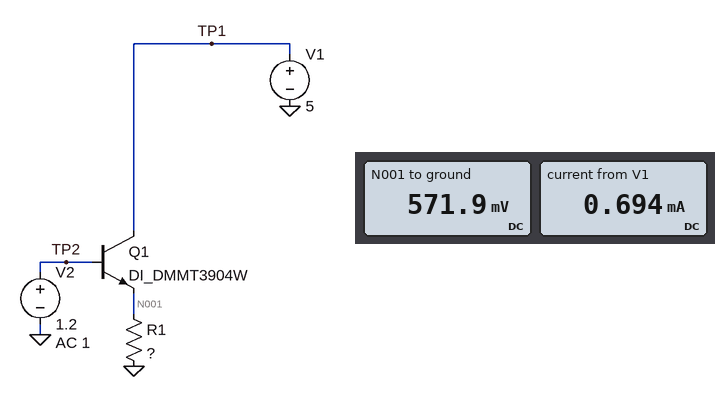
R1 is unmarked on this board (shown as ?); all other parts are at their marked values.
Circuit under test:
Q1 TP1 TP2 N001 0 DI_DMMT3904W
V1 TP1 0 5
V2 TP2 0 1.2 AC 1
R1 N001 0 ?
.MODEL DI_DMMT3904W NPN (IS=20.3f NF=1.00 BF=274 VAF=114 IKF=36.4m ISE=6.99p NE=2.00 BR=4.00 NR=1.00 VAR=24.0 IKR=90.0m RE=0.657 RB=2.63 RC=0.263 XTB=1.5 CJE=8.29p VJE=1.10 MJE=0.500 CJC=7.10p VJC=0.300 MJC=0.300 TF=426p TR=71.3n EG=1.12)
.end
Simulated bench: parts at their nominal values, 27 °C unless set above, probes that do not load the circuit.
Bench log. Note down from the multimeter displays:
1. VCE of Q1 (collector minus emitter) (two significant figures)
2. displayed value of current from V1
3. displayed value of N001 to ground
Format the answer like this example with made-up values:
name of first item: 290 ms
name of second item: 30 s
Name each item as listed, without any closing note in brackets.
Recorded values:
VCE of Q1 (collector minus emitter): 4.4 V
displayed value of current from V1: 0.694 mA
displayed value of N001 to ground: 571.9 mV
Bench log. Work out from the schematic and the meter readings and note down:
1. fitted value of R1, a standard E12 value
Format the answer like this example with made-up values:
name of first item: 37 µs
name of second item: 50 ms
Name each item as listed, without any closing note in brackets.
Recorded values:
fitted value of R1, a standard E12 value: 820 Ω
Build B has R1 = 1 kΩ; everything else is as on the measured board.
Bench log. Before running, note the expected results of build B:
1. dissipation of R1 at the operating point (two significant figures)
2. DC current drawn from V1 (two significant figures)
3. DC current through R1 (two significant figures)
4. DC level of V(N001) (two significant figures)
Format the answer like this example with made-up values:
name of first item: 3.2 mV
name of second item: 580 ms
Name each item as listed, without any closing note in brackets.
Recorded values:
dissipation of R1 at the operating point: 330 µW
DC current drawn from V1: 570 µA
DC current through R1: 580 µA
DC level of V(N001): 580 mV
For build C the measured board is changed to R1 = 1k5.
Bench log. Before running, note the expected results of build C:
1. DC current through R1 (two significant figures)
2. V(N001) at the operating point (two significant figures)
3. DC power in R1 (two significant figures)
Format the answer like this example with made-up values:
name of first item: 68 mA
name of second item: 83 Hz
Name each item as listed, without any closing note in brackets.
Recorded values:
DC current through R1: 390 µA
V(N001) at the operating point: 590 mV
DC power in R1: 230 µW
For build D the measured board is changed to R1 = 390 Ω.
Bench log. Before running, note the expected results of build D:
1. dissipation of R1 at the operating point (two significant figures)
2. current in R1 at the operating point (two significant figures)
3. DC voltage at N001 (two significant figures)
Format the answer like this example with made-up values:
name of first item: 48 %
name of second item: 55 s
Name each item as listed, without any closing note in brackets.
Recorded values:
dissipation of R1 at the operating point: 780 µW
current in R1 at the operating point: 1.4 mA
DC voltage at N001: 550 mV
